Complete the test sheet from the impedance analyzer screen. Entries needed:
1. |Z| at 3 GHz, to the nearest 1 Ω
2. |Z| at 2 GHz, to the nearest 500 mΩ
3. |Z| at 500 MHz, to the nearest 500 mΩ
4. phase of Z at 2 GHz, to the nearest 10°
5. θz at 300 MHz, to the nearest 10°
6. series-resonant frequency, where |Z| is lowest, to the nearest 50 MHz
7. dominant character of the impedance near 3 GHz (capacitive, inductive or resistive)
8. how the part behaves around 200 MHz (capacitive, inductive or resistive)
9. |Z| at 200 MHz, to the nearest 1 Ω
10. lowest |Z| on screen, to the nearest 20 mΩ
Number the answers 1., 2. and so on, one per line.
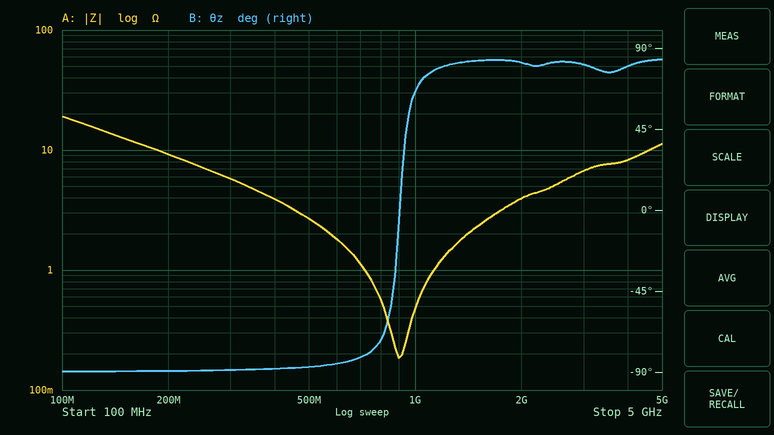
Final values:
1. 7 Ω
2. 4.0 Ω
3. 2.5 Ω
4. 80°
5. -90°
6. 900 MHz
7. inductive
8. capacitive
9. 9 Ω
10. 180 mΩ
